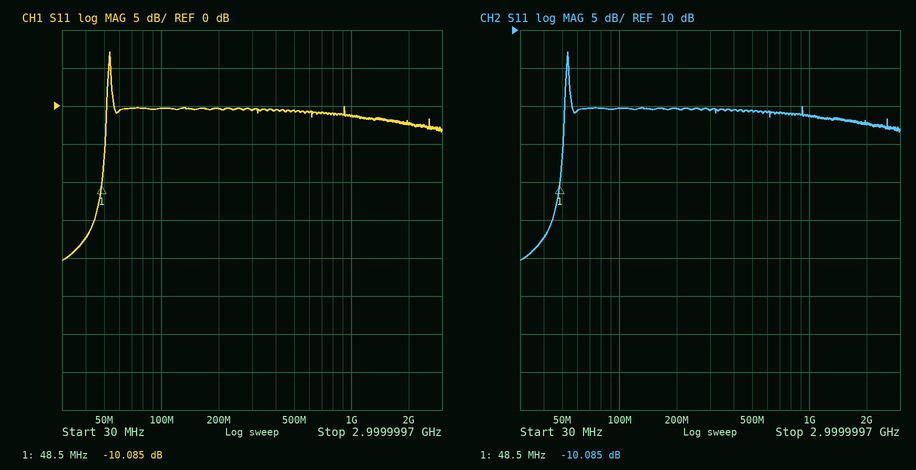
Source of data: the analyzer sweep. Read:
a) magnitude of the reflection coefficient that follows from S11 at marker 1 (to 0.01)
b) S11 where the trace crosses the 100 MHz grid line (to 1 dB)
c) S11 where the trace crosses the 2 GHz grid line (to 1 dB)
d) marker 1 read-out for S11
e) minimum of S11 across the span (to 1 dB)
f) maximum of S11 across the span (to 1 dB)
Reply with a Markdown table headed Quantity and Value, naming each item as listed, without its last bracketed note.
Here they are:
| Quantity | Value |
|---|---|
| magnitude of the reflection coefficient that follows from S11 at marker 1 | 0.31 |
| S11 where the trace crosses the 100 MHz grid line | 0 dB |
| S11 where the trace crosses the 2 GHz grid line | -2 dB |
| marker 1 read-out for S11 | -10.085 dB |
| minimum of S11 across the span | -20 dB |
| maximum of S11 across the span | 7 dB |
